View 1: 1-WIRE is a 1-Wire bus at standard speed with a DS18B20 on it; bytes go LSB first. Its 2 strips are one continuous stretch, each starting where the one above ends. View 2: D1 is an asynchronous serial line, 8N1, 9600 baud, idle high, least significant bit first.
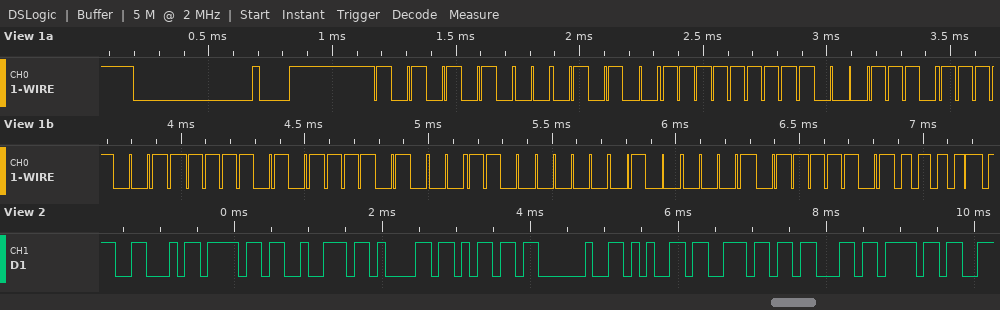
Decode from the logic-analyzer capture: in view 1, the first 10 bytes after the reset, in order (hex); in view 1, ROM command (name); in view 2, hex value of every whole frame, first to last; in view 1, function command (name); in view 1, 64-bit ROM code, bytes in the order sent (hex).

55 28 FF 71 CF AF 17 03 82 BE
Match ROM
46 6F 72 61 6D 20 65 6E 63 6F
Read Scratchpad
28 FF 71 CF AF 17 03 82
